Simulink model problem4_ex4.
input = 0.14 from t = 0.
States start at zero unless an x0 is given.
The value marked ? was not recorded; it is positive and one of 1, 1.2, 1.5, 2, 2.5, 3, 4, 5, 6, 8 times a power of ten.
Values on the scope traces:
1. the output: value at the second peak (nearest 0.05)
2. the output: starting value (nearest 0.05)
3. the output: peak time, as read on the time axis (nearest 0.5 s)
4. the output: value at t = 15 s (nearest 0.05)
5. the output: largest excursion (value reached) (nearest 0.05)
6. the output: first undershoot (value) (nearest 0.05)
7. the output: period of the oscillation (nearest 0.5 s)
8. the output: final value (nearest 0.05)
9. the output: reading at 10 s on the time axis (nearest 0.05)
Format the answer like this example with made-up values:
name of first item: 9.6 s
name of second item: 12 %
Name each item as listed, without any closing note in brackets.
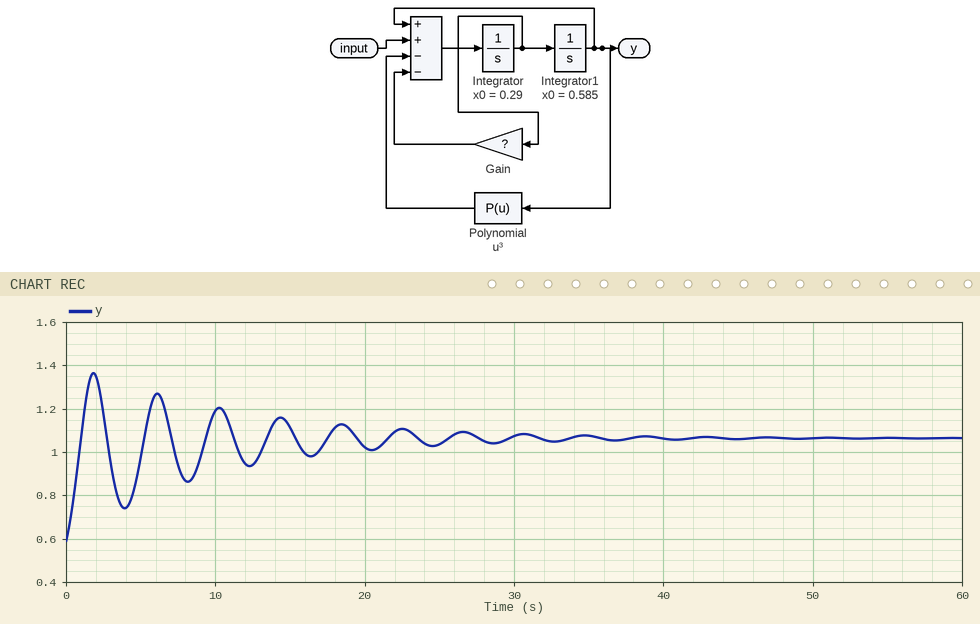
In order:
the output: value at the second peak: 1.25
the output: starting value: 0.60
the output: peak time, as read on the time axis: 2.0 s
the output: value at t = 15 s: 1.10
the output: largest excursion (value reached): 1.35
the output: first undershoot (value): 0.75
the output: period of the oscillation: 4.5 s
the output: final value: 1.05
the output: reading at 10 s on the time axis: 1.20
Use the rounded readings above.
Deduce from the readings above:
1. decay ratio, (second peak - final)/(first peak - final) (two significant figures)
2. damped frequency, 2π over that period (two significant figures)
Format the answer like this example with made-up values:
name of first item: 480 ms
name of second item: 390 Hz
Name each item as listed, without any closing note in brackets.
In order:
decay ratio, (second peak - final)/(first peak - final): 0.67
damped frequency, 2π over that period: 1.4 rad/s
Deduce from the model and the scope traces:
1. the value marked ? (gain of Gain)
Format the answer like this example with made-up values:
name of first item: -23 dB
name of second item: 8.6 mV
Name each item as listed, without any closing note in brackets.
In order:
the value marked ?: 0.2
